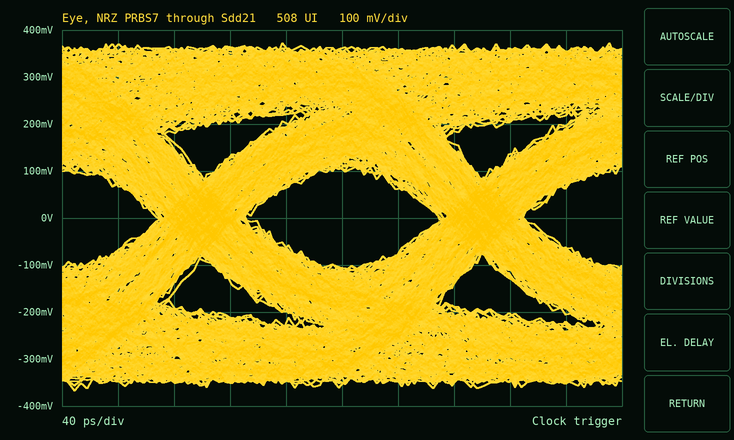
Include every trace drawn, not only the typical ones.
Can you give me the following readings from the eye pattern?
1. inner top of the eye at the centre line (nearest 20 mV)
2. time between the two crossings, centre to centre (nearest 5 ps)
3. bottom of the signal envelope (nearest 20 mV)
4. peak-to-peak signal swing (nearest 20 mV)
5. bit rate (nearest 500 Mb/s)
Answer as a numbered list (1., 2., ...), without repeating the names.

1. 100 mV
2. 200 ps
3. -360 mV
4. 740 mV
5. 5.0 Gb/s
